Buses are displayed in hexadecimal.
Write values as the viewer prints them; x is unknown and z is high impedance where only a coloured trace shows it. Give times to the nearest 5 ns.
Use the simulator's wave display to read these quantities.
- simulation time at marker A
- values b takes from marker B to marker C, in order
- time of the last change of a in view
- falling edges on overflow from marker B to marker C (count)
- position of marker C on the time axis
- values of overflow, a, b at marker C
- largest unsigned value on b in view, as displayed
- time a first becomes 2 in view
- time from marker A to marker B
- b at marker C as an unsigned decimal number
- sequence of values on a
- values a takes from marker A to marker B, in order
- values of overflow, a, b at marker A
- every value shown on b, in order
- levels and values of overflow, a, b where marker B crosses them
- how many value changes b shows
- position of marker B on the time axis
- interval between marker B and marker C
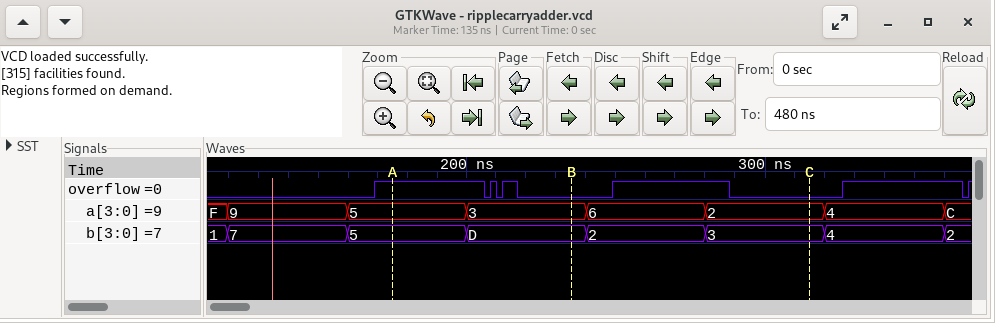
175 ns
D, 2, 3
360 ns
1
315 ns
overflow=0, a=2, b=3
D
280 ns
60 ns
3
F, 9, 5, 3, 6, 2, 4, C
5, 3
overflow=1, a=5, b=5
1, 7, 5, D, 2, 3, 4, 2
overflow=0, a=3, b=D
7
235 ns
80 ns
